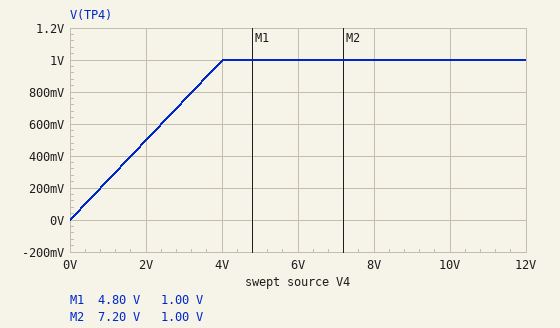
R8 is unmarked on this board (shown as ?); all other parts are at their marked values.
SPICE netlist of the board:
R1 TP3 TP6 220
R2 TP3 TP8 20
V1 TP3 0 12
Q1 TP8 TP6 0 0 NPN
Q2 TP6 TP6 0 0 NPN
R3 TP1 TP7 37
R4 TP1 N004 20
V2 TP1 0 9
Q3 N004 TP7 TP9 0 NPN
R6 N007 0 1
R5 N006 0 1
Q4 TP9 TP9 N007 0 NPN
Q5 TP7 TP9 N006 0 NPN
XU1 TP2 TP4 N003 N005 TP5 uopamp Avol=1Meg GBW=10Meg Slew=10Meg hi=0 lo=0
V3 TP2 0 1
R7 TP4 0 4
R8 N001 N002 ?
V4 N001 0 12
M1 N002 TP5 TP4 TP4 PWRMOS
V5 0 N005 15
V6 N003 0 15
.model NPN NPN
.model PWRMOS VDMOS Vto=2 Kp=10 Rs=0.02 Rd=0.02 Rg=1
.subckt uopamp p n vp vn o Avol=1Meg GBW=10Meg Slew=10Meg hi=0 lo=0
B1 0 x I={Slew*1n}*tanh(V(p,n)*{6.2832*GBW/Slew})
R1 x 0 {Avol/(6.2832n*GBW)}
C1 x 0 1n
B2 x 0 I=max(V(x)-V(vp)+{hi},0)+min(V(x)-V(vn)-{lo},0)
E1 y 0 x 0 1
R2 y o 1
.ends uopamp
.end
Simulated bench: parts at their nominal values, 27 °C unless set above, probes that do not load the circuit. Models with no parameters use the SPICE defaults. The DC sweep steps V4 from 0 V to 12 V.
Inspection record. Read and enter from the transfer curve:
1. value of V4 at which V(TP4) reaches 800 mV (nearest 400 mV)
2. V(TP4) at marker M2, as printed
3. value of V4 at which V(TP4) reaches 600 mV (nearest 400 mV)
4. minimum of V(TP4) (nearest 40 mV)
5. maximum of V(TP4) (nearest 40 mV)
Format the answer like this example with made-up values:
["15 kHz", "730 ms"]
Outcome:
["3.2 V", "1.00 V", "2.4 V", "0 V", "1.00 V"]
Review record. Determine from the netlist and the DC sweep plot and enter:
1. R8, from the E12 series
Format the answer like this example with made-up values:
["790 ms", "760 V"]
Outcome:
["12 Ω"]
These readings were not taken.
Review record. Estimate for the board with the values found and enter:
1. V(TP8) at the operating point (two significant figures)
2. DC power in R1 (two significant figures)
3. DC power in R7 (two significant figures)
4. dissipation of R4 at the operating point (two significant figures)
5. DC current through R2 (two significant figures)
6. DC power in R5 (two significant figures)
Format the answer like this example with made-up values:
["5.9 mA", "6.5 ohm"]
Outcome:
["11 V", "560 mW", "250 mW", "710 mW", "50 mA", "36 mW"]
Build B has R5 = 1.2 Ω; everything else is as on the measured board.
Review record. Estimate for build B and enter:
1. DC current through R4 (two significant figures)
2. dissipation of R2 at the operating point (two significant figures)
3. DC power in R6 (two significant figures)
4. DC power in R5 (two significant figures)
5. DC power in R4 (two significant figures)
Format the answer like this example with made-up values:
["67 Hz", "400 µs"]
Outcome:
["220 mA", "49 mW", "49 mW", "42 mW", "970 mW"]
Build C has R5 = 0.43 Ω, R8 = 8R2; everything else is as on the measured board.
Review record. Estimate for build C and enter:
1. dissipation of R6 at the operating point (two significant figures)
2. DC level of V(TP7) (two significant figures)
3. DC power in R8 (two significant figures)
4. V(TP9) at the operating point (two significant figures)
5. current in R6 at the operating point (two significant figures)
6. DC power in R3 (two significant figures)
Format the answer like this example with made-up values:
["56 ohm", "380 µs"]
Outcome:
["10 mW", "1.9 V", "510 mW", "990 mV", "100 mA", "1.4 W"]
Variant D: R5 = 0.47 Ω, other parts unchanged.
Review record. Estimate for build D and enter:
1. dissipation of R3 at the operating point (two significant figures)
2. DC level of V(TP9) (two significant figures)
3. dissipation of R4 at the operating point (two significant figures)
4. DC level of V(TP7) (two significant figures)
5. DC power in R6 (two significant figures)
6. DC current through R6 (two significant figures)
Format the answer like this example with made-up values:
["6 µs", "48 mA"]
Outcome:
["1.4 W", "1.0 V", "230 mW", "1.9 V", "11 mW", "110 mA"]
